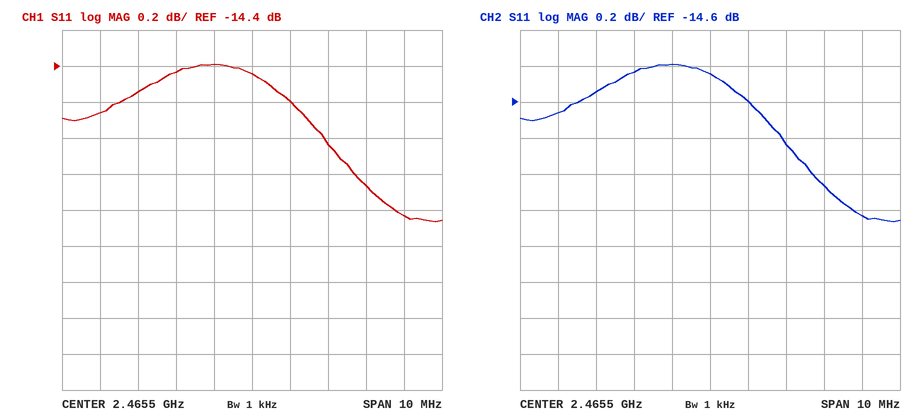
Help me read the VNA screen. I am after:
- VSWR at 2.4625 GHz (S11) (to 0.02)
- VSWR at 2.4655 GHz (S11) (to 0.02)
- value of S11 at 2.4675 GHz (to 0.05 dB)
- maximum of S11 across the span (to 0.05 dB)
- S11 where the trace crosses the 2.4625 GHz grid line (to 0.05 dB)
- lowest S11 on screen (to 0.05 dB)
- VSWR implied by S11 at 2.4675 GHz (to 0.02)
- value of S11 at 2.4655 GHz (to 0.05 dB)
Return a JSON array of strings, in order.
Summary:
["1.46", "1.46", "-14.85 dB", "-14.40 dB", "-14.55 dB", "-15.25 dB", "1.44", "-14.45 dB"]
